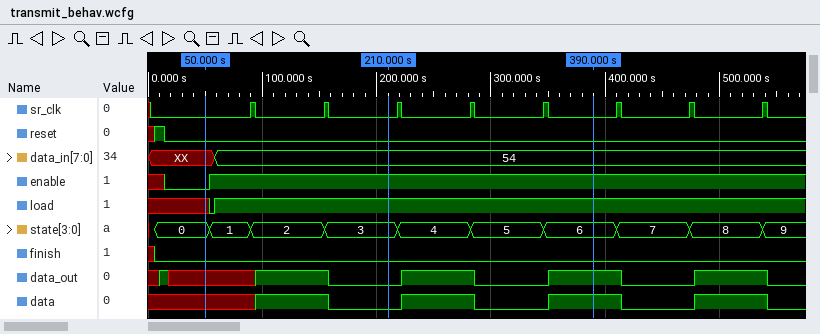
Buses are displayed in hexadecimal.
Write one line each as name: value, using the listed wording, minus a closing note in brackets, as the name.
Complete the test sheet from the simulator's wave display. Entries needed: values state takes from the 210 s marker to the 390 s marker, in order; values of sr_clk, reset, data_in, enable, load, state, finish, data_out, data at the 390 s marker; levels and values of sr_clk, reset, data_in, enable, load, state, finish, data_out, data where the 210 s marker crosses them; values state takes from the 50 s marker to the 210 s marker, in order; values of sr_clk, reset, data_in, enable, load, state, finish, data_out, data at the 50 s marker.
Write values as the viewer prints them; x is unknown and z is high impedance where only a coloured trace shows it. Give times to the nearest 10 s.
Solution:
values state takes from the 210 s marker to the 390 s marker, in order: 3, 4, 5, 6
values of sr_clk, reset, data_in, enable, load, state, finish, data_out, data at the 390 s marker: sr_clk=0, reset=0, data_in=54, enable=1, load=1, state=6, finish=0, data_out=1, data=1
levels and values of sr_clk, reset, data_in, enable, load, state, finish, data_out, data where the 210 s marker crosses them: sr_clk=0, reset=0, data_in=54, enable=1, load=1, state=3, finish=0, data_out=0, data=0
values state takes from the 50 s marker to the 210 s marker, in order: 0, 1, 2, 3
values of sr_clk, reset, data_in, enable, load, state, finish, data_out, data at the 50 s marker: sr_clk=0, reset=0, data_in=XX, enable=0, load=x, state=0, finish=0, data_out=x, data=x
